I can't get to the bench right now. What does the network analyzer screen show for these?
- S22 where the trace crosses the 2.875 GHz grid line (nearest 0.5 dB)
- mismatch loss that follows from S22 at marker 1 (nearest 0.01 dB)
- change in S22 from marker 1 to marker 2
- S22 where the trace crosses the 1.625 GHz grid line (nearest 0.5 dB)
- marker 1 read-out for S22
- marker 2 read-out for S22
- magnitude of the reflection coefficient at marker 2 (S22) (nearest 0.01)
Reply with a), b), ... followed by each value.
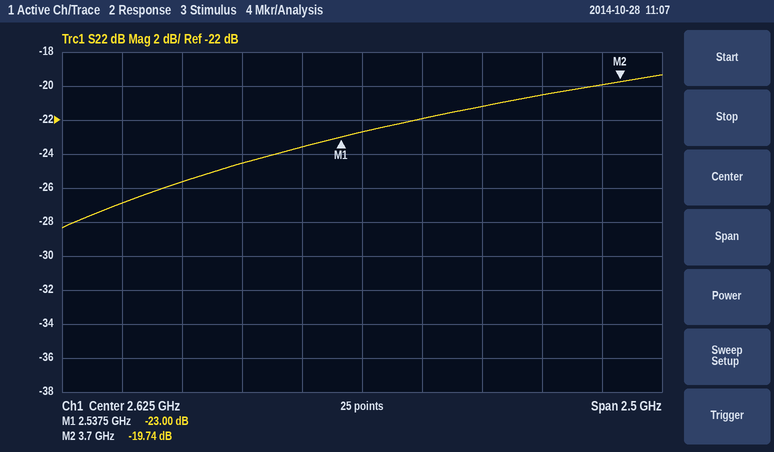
a) -22.0 dB
b) 0.02 dB
c) 3.26 dB
d) -27.0 dB
e) -23.00 dB
f) -19.74 dB
g) 0.10
